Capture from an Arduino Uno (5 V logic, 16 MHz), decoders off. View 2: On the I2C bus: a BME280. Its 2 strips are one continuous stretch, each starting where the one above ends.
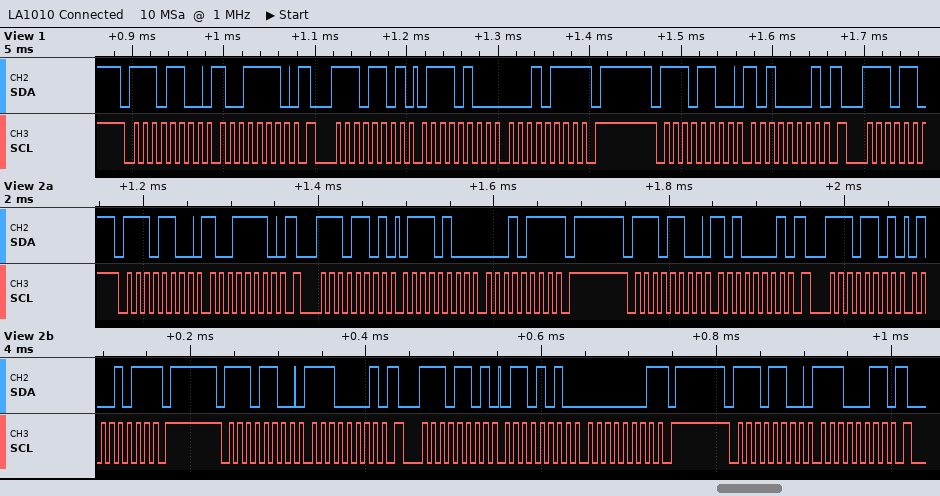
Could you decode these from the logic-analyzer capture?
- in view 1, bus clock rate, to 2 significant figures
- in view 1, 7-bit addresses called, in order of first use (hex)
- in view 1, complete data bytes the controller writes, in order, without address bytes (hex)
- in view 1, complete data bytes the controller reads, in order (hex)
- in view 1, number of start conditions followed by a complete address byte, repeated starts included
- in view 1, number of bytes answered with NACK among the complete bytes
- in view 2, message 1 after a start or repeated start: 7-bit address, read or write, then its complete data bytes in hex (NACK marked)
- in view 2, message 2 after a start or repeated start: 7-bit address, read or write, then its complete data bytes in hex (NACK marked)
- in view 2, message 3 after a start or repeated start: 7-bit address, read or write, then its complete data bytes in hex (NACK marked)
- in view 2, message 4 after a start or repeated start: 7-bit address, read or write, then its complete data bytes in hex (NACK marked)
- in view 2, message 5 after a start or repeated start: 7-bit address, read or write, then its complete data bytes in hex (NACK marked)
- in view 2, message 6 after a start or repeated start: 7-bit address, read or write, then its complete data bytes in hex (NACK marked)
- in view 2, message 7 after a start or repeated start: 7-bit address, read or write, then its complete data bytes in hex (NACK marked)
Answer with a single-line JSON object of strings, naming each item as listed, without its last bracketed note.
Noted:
{"in view 1, bus clock rate, to 2 significant figures": "100 kHz", "in view 1, 7-bit addresses called, in order of first use": "0x76", "in view 1, complete data bytes the controller writes, in order, without address bytes": "9E A1", "in view 1, complete data bytes the controller reads, in order": "74 17", "in view 1, number of start conditions followed by a complete address byte, repeated starts included": "3", "in view 1, number of bytes answered with NACK among the complete bytes": "1", "in view 2, message 1 after a start or repeated start: 7-bit address, read or write, then its complete data bytes in hex": "0x76 write: 9E", "in view 2, message 2 after a start or repeated start: 7-bit address, read or write, then its complete data bytes in hex": "0x76 read: 74 17 NACK", "in view 2, message 3 after a start or repeated start: 7-bit address, read or write, then its complete data bytes in hex": "0x76 write: A1", "in view 2, message 4 after a start or repeated start: 7-bit address, read or write, then its complete data bytes in hex": "0x76 read: 4B NACK", "in view 2, message 5 after a start or repeated start: 7-bit address, read or write, then its complete data bytes in hex": "0x76 write: E1", "in view 2, message 6 after a start or repeated start: 7-bit address, read or write, then its complete data bytes in hex": "0x76 read: 6A 01 NACK", "in view 2, message 7 after a start or repeated start: 7-bit address, read or write, then its complete data bytes in hex": "0x76 write: E3"}
